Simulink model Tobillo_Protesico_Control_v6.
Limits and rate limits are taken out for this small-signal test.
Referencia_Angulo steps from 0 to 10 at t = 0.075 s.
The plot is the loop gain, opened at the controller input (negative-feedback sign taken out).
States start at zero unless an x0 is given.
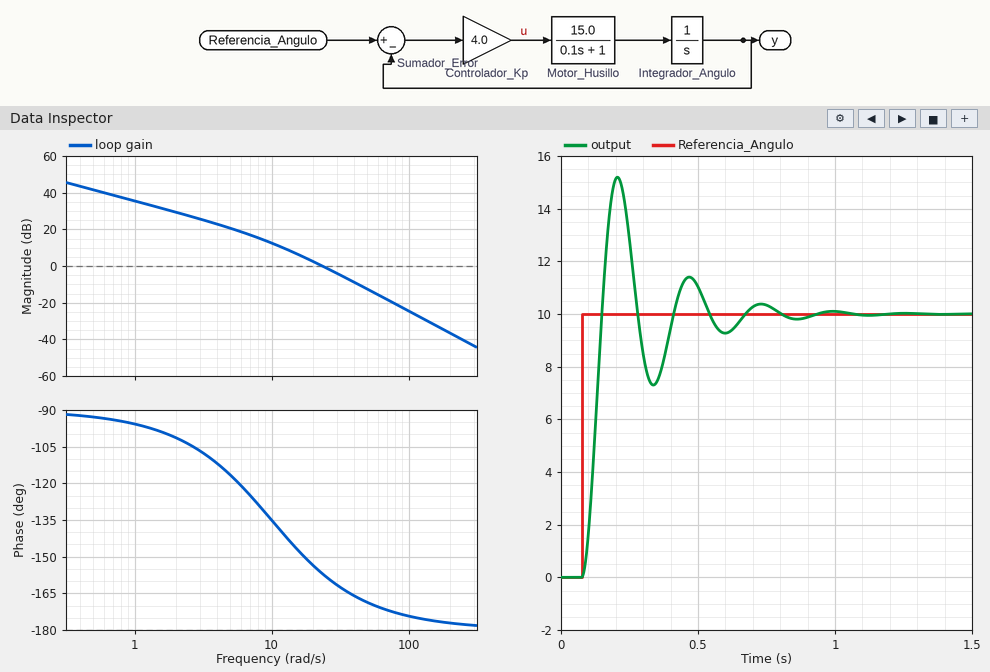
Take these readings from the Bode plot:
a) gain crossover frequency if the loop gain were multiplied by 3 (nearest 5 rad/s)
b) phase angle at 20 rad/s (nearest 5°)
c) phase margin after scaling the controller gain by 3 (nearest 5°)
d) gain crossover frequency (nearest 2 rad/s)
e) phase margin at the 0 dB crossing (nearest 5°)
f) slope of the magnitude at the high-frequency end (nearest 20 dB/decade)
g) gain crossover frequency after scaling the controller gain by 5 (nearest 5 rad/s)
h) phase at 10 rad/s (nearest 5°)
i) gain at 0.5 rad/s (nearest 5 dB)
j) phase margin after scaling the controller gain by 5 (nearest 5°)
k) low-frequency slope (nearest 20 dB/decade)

40 rad/s
-155°
15°
24 rad/s
25°
-40 dB/decade
55 rad/s
-135°
40 dB
10°
-20 dB/decade
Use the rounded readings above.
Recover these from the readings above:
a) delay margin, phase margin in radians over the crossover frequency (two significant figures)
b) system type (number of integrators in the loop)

0.018 s
1
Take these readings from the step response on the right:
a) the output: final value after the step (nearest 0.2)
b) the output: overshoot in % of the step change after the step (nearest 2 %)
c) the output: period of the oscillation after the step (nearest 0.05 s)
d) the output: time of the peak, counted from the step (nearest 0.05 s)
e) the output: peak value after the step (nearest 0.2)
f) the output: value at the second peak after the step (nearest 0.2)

10.0
52 %
0.25 s
0.15 s
15.2
11.4
